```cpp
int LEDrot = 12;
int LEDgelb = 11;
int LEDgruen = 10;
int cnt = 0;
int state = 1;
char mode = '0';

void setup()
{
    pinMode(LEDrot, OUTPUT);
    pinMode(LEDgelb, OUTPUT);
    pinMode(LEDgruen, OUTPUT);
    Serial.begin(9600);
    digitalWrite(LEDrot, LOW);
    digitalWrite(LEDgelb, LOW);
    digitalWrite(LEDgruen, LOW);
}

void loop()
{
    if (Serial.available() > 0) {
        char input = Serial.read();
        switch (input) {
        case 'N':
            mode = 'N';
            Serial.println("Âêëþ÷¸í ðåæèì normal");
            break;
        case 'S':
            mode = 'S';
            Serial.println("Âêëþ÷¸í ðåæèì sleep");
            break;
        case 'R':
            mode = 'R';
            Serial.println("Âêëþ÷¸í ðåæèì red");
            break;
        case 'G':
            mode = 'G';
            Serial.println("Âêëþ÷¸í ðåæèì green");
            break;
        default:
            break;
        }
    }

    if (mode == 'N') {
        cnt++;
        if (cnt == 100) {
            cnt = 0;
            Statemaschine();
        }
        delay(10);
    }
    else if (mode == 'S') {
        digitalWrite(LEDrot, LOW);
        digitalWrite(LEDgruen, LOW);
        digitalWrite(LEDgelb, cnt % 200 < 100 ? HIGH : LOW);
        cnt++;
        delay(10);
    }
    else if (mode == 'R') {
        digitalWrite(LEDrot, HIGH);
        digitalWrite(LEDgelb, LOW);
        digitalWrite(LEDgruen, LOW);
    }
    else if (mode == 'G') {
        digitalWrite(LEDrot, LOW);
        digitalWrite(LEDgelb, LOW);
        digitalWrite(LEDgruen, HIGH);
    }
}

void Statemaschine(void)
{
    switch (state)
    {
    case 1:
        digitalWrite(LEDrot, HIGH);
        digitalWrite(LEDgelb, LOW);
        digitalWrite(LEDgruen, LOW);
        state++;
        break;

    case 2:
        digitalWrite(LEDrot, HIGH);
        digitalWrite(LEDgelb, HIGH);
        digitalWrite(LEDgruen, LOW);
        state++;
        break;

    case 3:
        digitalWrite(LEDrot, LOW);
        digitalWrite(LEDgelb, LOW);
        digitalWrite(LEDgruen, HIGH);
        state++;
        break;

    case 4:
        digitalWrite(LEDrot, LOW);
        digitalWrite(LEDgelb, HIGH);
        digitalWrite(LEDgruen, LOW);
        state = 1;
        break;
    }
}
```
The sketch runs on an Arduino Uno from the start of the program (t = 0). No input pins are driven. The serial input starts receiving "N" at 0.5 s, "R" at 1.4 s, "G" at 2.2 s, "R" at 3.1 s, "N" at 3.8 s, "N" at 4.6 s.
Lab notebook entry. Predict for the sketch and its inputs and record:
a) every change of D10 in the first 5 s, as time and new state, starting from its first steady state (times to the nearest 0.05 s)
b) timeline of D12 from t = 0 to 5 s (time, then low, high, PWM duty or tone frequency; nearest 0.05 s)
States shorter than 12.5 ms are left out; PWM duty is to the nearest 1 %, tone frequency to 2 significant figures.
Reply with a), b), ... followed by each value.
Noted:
a) 0 s low; 2.2 s high; 3.1 s low
b) 0 s low; 1.4 s high; 2.2 s low; 3.1 s high
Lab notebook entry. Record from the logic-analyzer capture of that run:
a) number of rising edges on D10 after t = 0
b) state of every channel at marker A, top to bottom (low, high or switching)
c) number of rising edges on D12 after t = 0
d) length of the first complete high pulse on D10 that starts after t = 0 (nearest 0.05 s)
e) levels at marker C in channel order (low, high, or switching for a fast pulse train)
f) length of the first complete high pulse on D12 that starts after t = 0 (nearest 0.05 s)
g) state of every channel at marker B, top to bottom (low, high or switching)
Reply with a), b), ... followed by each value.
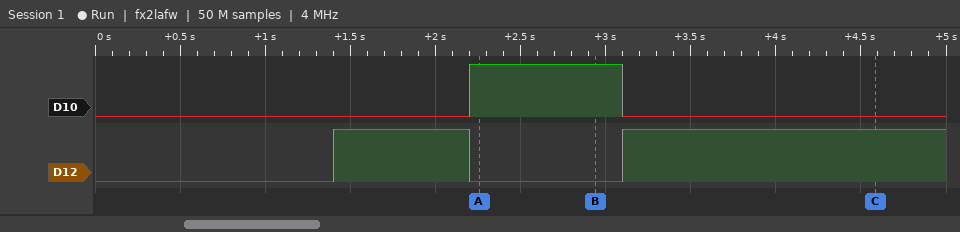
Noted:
a) 1
b) D10 high, D12 low
c) 2
d) 0.90 s
e) D10 low, D12 high
f) 0.80 s
g) D10 high, D12 low
